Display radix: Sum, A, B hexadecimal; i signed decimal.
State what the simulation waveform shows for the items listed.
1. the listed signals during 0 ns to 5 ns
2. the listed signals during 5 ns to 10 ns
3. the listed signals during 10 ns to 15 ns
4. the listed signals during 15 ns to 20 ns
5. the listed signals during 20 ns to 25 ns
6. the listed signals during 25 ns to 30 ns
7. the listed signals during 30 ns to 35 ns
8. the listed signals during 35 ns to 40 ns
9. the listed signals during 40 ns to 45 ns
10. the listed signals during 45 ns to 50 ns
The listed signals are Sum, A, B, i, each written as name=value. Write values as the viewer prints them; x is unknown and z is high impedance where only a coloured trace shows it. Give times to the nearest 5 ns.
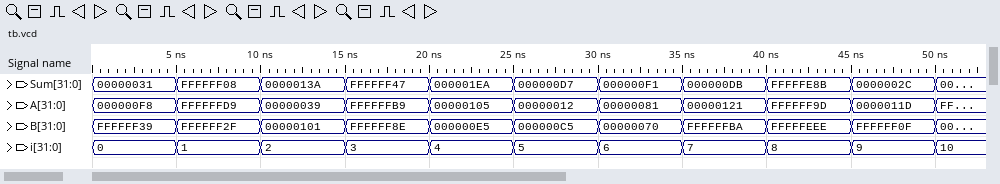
Sum=00000031, A=000000F8, B=FFFFFF39, i=0
Sum=FFFFFF08, A=FFFFFFD9, B=FFFFFF2F, i=1
Sum=0000013A, A=00000039, B=00000101, i=2
Sum=FFFFFF47, A=FFFFFFB9, B=FFFFFF8E, i=3
Sum=000001EA, A=00000105, B=000000E5, i=4
Sum=000000D7, A=00000012, B=000000C5, i=5
Sum=000000F1, A=00000081, B=00000070, i=6
Sum=000000DB, A=00000121, B=FFFFFFBA, i=7
Sum=FFFFFE8B, A=FFFFFF9D, B=FFFFFEEE, i=8
Sum=0000002C, A=0000011D, B=FFFFFF0F, i=9
